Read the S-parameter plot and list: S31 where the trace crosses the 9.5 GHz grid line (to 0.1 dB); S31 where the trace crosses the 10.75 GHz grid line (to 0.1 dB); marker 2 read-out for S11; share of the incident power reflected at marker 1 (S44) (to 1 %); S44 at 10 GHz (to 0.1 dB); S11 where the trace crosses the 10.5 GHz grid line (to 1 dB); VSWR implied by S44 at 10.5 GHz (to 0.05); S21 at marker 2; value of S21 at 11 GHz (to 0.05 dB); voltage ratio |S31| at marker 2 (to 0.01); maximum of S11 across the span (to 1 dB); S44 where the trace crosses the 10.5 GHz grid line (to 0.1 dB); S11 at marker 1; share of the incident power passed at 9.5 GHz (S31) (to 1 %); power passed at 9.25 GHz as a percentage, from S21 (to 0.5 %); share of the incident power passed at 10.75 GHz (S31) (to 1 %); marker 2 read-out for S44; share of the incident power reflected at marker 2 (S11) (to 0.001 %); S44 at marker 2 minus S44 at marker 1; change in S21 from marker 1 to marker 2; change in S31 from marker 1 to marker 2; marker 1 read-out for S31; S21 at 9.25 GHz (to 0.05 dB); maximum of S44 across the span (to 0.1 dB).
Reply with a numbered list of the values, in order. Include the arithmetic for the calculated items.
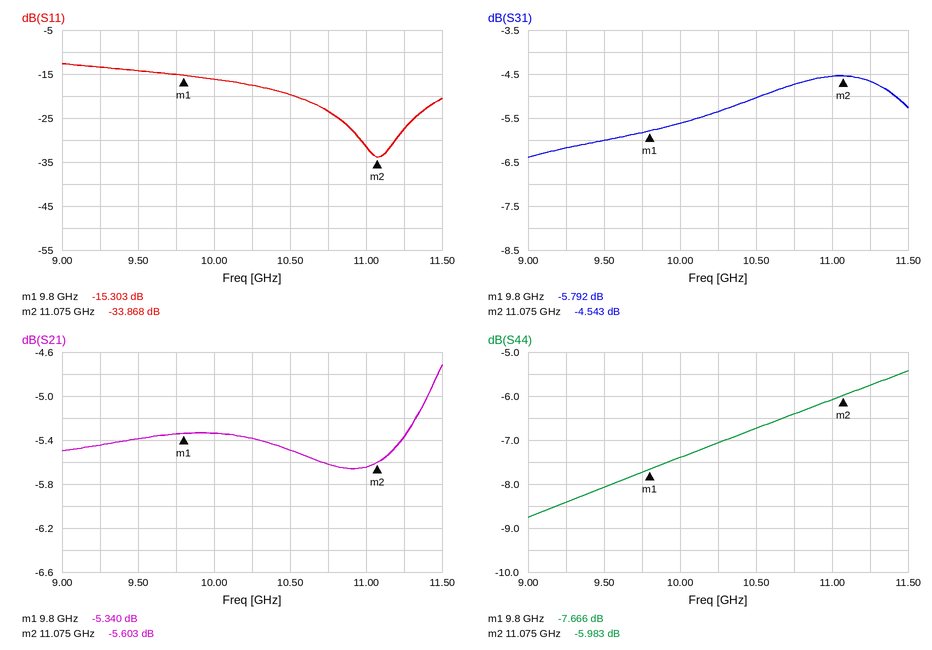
1. -6.0 dB
2. -4.7 dB
3. -33.868 dB
4. 10^(-7.666/10) ≈ 17 %
5. -7.4 dB
6. -20 dB
7. |Γ| = 10^(-6.7/20) = 0.4624; VSWR = (1 + 0.4624)/(1 − 0.4624) ≈ 2.72, so 2.70 to the nearest 0.05
8. -5.603 dB
9. -5.65 dB
10. 10^(-4.543/20) ≈ 0.59
11. -13 dB
12. -6.7 dB
13. -15.303 dB
14. 10^(-6/10) ≈ 25 %
15. 10^(-5.45/10) ≈ 28.5 %
16. 10^(-4.7/10) ≈ 34 %
17. -5.983 dB
18. 10^(-33.868/10) ≈ 0.041 %
19. -5.983 − (-7.666) = 1.683 dB
20. -5.603 − (-5.34) = -0.263 dB
21. -4.543 − (-5.792) = 1.249 dB
22. -5.792 dB
23. -5.45 dB
24. -5.4 dB
